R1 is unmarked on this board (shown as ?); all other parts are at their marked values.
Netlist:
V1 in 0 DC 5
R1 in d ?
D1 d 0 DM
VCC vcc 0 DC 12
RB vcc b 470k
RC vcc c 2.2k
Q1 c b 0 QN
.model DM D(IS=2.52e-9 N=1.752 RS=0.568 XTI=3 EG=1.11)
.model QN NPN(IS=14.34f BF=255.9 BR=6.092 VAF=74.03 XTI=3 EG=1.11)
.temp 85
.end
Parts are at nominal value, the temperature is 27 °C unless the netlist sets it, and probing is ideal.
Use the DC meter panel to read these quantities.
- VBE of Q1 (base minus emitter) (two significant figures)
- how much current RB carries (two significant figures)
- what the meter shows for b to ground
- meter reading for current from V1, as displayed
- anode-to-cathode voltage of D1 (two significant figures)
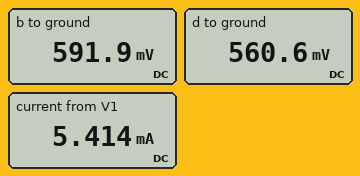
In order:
590 mV
24 µA
591.9 mV
5.414 mA
560 mV
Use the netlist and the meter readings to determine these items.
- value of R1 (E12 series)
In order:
820 Ω
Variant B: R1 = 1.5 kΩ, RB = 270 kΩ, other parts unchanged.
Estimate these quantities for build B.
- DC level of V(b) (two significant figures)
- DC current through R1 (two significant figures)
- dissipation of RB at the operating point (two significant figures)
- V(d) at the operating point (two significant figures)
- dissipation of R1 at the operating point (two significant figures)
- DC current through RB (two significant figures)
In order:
590 mV
3.0 mA
480 µW
530 mV
13 mW
42 µA
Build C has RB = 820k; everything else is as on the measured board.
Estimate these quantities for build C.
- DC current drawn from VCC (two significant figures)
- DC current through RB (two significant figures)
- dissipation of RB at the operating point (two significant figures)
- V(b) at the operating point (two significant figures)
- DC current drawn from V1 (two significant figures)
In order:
3.7 mA
14 µA
160 µW
580 mV
5.4 mA
